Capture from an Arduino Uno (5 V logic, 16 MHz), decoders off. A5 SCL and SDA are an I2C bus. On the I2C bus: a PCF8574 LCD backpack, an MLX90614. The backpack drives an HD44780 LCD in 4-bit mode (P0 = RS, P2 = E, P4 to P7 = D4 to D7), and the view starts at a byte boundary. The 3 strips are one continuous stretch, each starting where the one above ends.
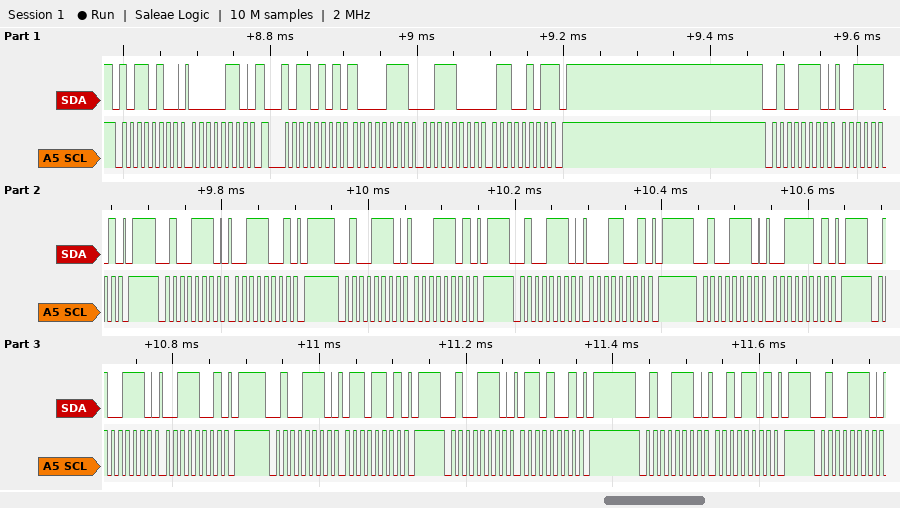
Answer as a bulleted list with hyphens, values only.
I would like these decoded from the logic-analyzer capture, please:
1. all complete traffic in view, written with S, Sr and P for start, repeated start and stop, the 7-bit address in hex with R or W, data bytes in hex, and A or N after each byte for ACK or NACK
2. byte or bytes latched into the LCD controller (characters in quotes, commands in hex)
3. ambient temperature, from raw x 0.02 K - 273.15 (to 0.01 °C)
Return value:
- S 5AW A 06 A Sr 5AR A 87 A 38 A 65 N P S 27W A 3D A P S 27W A 39 A P S 27W A 1D A P S 27W A 19 A P S 27W A 3D A P S 27W A 39 A P S 27W A 6D A P S 27W A 69 A P S 27W A 2D A P S 27W A
- '1' '6'
- 16.27 °C
